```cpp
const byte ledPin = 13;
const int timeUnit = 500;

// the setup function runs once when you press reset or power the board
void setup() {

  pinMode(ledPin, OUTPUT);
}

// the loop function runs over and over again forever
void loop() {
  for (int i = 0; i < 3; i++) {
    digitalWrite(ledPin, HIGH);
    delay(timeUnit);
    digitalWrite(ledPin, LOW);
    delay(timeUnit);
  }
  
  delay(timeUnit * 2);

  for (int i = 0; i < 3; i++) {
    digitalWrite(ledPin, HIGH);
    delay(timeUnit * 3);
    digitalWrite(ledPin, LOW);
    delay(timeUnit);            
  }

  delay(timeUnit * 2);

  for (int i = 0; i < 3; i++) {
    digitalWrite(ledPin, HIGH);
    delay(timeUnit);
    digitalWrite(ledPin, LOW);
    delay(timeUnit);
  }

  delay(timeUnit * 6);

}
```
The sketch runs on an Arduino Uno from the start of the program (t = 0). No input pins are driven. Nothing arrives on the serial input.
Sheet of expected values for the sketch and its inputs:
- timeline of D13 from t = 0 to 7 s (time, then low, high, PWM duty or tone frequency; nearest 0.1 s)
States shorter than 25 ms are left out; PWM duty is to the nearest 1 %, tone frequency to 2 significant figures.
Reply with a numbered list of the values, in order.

1. 0 s high; 0.5 s low; 1 s high; 1.5 s low; 2 s high; 2.5 s low; 4 s high; 5.5 s low; 6 s high
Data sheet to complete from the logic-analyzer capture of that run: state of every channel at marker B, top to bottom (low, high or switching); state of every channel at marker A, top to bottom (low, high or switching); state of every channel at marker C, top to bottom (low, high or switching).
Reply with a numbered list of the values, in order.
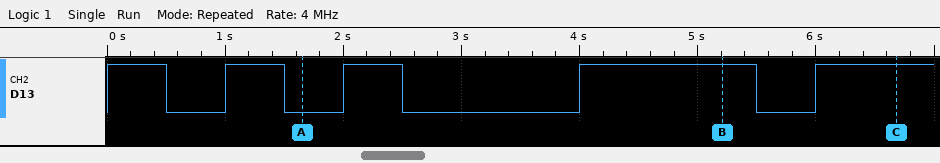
1. D13 high
2. D13 low
3. D13 high
